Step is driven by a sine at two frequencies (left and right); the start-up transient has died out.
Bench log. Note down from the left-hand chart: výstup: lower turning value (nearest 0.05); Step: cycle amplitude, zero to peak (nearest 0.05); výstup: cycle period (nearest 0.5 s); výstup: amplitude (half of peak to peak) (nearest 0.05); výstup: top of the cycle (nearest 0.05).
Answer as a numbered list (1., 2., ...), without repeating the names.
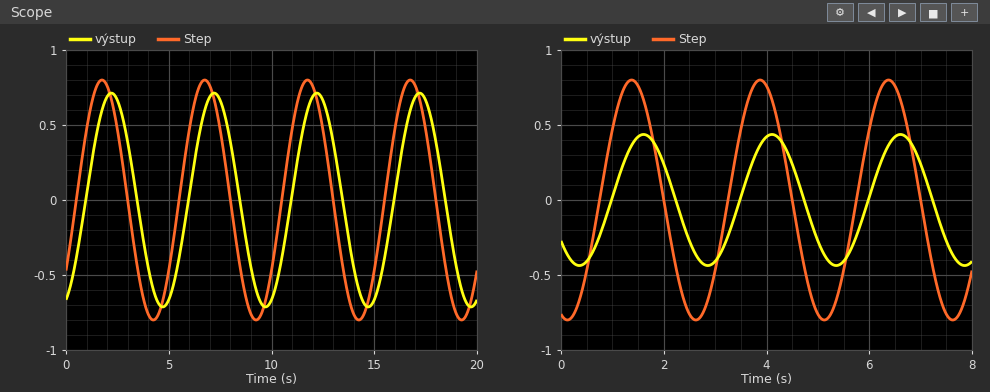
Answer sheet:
1. -0.70
2. 0.80
3. 5.0 s
4. 0.70
5. 0.70
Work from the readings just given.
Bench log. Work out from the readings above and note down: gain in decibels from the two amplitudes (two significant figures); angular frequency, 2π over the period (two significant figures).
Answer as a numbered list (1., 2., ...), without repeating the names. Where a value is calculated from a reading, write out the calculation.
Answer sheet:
1. 20 log10(0.7 / 0.8) = -1.2 dB
2. 2π / 5 = 1.3 rad/s
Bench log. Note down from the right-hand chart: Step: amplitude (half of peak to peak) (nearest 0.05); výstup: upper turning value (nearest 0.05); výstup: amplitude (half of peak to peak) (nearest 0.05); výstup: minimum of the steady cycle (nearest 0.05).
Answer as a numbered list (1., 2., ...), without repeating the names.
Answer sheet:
1. 0.80
2. 0.45
3. 0.45
4. -0.45
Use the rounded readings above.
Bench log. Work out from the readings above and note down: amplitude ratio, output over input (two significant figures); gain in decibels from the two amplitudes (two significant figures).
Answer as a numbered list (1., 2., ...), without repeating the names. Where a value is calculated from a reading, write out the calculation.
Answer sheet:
1. 0.45 / 0.8 = 0.56
2. 20 log10(0.45 / 0.8) = -5.0 dB
